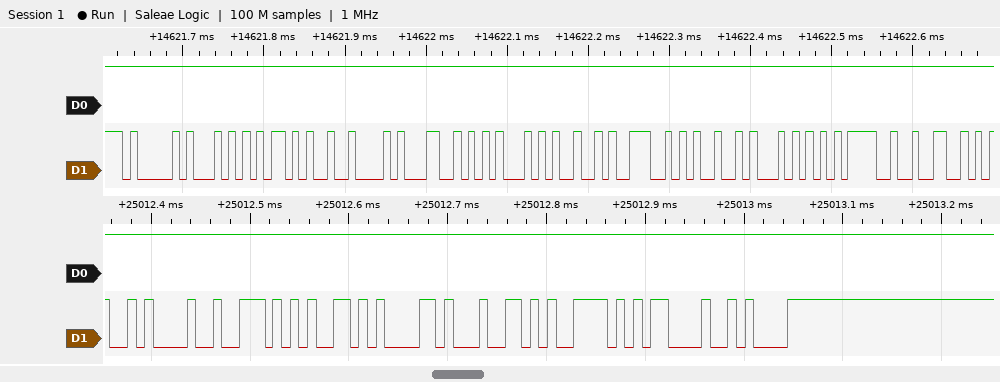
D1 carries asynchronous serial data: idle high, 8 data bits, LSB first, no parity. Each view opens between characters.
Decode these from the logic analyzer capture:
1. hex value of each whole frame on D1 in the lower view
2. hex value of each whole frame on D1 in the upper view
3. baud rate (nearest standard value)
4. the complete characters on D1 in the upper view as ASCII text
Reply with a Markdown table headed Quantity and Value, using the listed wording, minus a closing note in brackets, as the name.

| Quantity | Value |
|---|---|
| hex value of each whole frame on D1 in the lower view | 0A, 72, 65, 61, 64, 79, 0D, 0A |
| hex value of each whole frame on D1 in the upper view | 41, 54, 2B, 42, 4C, 45, 49, 4E, 49, 54, 3D, 32 |
| baud rate | 115200 baud |
| the complete characters on D1 in the upper view as ASCII text | "AT+BLEINIT=2" |
